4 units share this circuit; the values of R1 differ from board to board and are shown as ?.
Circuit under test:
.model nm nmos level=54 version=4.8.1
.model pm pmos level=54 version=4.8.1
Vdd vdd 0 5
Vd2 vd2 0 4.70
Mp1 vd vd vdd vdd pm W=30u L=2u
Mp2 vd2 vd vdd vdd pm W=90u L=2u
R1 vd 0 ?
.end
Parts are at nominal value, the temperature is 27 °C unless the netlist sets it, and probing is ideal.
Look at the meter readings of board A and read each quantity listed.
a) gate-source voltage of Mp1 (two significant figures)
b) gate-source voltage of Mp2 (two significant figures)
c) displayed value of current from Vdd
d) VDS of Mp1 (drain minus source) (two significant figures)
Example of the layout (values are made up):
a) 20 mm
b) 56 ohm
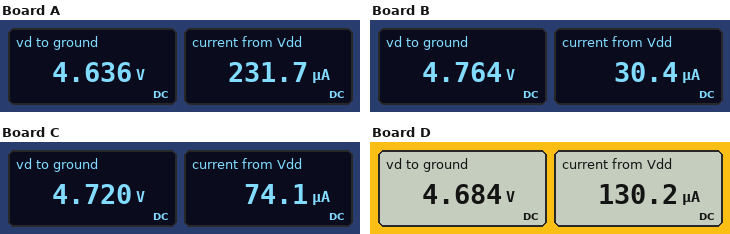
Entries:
a) -360 mV
b) -360 mV
c) 231.7 µA
d) -360 mV
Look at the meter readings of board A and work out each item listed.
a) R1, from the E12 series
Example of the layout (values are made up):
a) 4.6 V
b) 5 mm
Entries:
a) 82 kΩ
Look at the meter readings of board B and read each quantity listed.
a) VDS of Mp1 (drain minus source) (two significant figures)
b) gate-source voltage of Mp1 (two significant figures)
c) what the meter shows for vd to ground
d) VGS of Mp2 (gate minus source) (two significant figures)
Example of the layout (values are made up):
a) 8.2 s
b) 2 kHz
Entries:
a) -240 mV
b) -240 mV
c) 4.764 V
d) -240 mV
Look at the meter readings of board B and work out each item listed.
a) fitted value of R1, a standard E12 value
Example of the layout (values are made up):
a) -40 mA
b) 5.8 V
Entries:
a) 680 kΩ
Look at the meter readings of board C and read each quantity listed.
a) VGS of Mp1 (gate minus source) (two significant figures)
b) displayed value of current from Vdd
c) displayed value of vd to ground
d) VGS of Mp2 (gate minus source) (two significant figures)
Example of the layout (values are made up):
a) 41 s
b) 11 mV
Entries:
a) -280 mV
b) 74.1 µA
c) 4.720 V
d) -280 mV
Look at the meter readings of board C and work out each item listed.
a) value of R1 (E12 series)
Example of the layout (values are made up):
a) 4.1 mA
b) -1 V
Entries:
a) 270 kΩ
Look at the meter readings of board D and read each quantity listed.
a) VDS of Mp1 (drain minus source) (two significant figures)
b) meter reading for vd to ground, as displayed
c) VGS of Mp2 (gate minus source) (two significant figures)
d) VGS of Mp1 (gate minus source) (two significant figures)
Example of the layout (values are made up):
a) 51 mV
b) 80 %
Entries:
a) -320 mV
b) 4.684 V
c) -320 mV
d) -320 mV
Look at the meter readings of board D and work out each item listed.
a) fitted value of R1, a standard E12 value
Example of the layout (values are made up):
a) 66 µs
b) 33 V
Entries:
a) 150 kΩ
